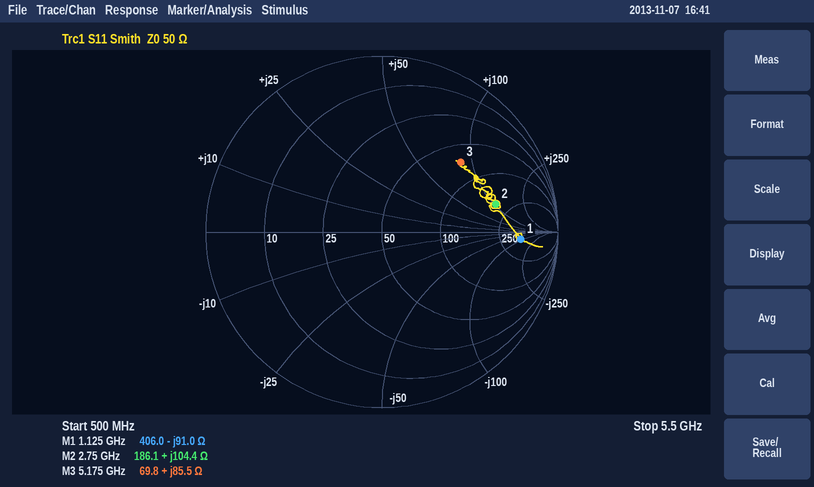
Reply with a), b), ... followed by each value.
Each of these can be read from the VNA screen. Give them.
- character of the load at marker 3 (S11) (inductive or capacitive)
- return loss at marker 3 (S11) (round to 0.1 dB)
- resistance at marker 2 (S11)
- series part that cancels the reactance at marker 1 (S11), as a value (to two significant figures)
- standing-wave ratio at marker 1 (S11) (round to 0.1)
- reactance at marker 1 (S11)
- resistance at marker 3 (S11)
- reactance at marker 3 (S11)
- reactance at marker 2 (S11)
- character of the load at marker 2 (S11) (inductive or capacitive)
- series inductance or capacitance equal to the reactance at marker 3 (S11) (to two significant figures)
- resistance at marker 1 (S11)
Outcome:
a) inductive
b) 4.5 dB
c) 186.1 Ω
d) 13 nH
e) 8.5
f) -91.0 Ω
g) 69.8 Ω
h) +85.5 Ω
i) +104.4 Ω
j) inductive
k) 2.6 nH
l) 406.0 Ω
